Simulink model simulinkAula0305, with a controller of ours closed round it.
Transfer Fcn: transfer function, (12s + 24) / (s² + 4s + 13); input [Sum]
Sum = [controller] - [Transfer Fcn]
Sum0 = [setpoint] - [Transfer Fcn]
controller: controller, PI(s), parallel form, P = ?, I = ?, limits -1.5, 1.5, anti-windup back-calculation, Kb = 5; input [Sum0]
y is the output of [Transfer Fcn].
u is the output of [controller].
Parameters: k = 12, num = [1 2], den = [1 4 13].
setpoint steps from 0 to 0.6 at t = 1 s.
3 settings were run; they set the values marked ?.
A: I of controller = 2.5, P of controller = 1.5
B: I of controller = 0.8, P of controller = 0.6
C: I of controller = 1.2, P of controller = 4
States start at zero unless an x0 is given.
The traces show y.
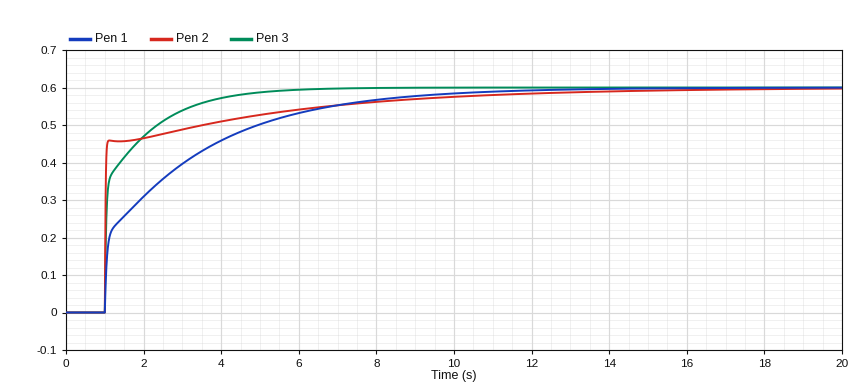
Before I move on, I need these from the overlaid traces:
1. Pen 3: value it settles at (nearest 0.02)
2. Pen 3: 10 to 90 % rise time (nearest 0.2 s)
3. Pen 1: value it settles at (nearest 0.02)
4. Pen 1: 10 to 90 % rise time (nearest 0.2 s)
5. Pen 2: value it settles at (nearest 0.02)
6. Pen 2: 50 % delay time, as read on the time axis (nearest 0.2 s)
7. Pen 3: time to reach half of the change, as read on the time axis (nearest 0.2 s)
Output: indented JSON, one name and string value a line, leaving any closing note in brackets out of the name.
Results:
{
  "Pen 3: value it settles at": "0.60",
  "Pen 3: 10 to 90 % rise time": "2.0 s",
  "Pen 1: value it settles at": "0.60",
  "Pen 1: 10 to 90 % rise time": "5.4 s",
  "Pen 2: value it settles at": "0.60",
  "Pen 2: 50 % delay time, as read on the time axis": "1.0 s",
  "Pen 3: time to reach half of the change, as read on the time axis": "1.0 s"
}
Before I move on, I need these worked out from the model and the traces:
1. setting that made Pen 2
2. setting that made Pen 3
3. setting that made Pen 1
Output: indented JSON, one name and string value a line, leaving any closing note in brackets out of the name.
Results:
{
  "setting that made Pen 2": "C",
  "setting that made Pen 3": "A",
  "setting that made Pen 1": "B"
}
